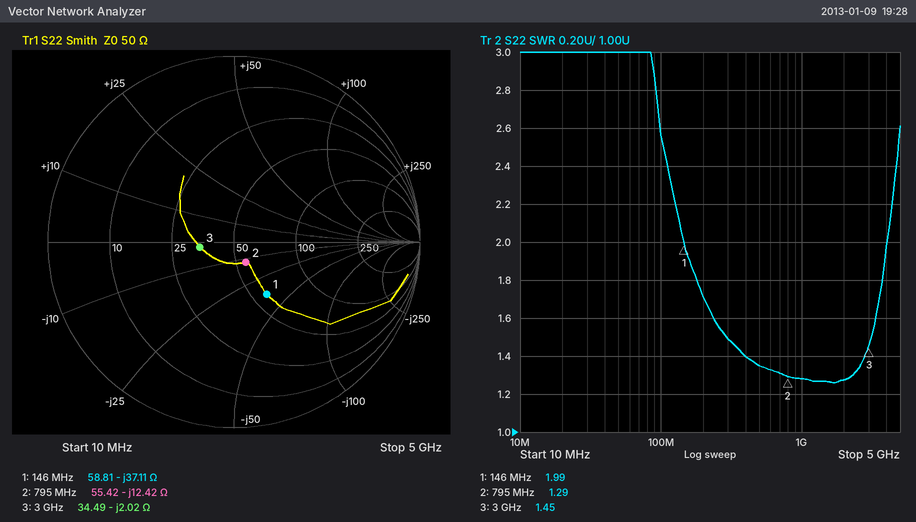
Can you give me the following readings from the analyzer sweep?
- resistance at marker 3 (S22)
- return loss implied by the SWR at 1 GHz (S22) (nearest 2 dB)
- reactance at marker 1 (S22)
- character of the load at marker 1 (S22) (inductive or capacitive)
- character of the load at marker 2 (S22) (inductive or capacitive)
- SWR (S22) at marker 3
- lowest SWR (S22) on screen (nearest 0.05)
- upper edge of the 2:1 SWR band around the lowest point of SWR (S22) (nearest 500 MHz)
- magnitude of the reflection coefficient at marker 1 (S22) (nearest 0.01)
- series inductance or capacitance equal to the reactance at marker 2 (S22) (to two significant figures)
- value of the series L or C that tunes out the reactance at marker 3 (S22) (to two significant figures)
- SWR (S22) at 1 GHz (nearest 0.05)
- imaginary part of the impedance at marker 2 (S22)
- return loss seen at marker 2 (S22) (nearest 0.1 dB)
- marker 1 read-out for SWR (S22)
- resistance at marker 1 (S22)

34.49 Ω
18 dB
-37.11 Ω
capacitive
capacitive
1.45
1.25
4.0 GHz
0.33
16 pF
110 pH
1.30
-12.42 Ω
17.9 dB
1.99
58.81 Ω
